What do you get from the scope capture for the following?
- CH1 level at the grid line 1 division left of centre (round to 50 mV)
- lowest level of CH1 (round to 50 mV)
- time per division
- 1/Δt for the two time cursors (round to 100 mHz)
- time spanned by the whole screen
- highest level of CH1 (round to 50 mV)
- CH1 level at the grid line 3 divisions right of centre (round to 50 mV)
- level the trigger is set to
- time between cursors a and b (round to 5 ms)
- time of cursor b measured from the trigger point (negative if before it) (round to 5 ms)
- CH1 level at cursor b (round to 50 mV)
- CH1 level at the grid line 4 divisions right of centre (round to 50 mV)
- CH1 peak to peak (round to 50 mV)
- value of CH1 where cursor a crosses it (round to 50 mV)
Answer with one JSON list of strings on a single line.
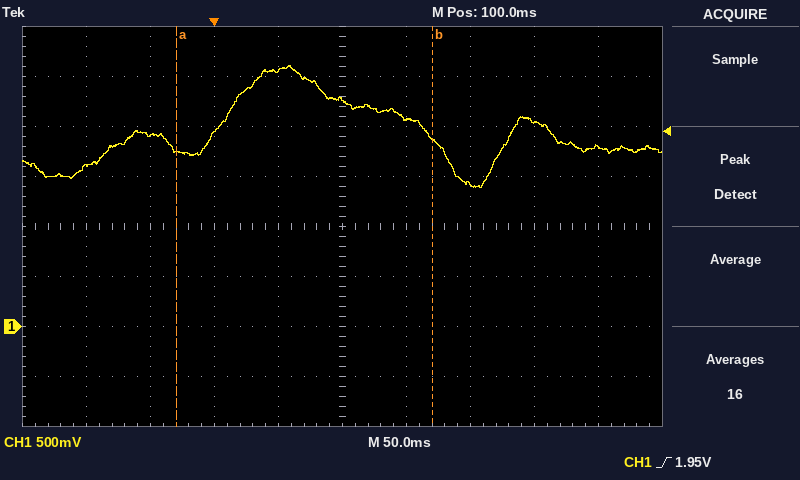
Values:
["2.55 V", "1.40 V", "50 ms", "5.0 Hz", "500 ms", "2.60 V", "2.05 V", "1.95 V", "200 ms", "+170 ms", "1.85 V", "1.80 V", "1.20 V", "1.75 V"]
